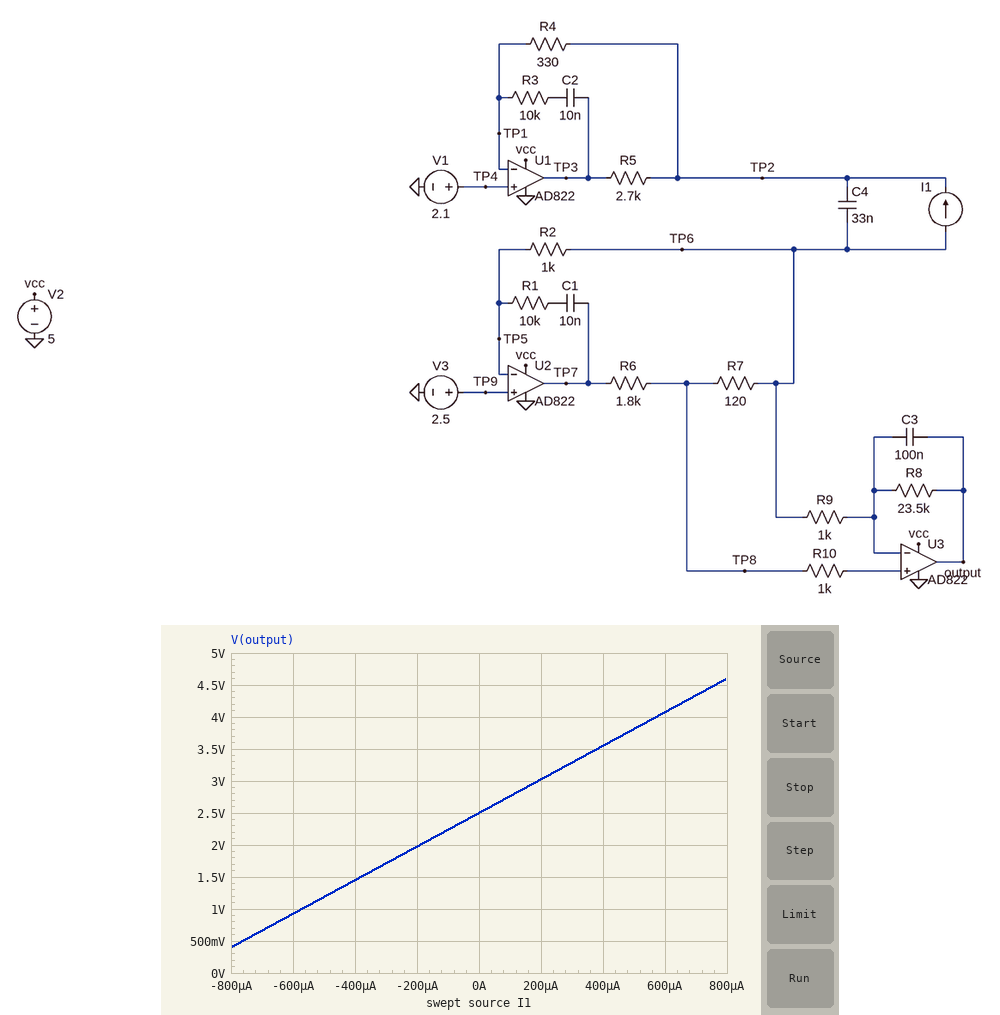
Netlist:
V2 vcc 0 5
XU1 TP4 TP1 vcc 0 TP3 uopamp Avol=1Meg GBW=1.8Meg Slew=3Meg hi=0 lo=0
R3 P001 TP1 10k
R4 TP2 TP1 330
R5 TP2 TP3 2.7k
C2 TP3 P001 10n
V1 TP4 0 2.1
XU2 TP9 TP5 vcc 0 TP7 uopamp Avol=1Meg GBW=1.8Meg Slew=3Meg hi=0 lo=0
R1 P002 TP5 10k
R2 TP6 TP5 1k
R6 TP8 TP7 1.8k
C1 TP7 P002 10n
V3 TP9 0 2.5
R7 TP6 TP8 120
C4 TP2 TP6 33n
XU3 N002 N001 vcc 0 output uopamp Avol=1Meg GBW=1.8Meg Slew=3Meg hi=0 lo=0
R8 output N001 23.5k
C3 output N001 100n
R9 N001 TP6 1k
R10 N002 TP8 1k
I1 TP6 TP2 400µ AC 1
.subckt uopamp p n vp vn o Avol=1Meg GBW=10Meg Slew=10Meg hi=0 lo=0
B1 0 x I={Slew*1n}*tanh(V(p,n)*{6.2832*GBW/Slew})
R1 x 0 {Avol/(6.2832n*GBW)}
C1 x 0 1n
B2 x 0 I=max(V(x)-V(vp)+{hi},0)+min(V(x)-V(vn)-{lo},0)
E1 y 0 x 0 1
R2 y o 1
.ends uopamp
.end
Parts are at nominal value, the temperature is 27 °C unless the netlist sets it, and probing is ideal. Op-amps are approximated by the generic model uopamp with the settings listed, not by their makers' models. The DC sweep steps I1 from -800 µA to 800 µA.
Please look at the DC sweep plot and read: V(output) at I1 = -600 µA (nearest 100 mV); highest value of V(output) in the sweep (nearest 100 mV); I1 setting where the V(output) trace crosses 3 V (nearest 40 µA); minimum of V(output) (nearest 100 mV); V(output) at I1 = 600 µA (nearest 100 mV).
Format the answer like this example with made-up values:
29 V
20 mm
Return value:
900 mV
4.6 V
200 µA
400 mV
4.1 V
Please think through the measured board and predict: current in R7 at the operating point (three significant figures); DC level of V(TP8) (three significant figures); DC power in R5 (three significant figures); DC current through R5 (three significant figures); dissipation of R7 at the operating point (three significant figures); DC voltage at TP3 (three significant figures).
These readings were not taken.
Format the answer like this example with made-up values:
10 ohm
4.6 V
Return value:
357 µA
2.54 V
432 µW
400 µA
15.3 µW
1.02 V
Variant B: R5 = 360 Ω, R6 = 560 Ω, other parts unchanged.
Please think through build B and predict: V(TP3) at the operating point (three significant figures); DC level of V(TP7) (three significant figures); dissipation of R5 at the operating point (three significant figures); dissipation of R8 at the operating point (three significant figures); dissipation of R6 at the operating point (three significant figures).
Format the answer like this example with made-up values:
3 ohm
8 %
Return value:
1.96 V
2.74 V
57.6 µW
43.2 µW
71.4 µW
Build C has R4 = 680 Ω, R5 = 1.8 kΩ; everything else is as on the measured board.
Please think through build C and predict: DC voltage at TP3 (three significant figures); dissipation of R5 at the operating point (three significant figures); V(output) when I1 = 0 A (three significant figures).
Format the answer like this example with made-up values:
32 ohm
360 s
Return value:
1.38 V
288 µW
2.50 V
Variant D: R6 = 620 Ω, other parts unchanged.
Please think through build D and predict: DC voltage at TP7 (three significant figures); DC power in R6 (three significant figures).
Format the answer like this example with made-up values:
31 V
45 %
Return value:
2.76 V
79.1 µW
